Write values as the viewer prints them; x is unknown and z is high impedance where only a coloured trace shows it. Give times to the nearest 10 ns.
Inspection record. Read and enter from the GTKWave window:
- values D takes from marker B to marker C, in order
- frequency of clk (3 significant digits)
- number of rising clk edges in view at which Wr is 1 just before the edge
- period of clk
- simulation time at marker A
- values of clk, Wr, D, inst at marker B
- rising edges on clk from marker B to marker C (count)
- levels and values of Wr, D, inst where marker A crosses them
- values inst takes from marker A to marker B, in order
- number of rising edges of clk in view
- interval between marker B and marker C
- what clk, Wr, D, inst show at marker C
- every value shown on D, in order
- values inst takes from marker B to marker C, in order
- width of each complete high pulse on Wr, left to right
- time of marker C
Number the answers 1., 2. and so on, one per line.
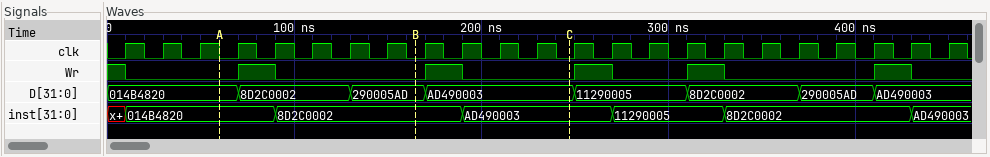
1. 290005AD, AD490003
2. 50.0 MHz
3. 6
4. 20 ns
5. 60 ns
6. clk=0, Wr=0, D=290005AD, inst=8D2C0002
7. 4
8. Wr=0, D=014B4820, inst=014B4820
9. 014B4820, 8D2C0002
10. 23
11. 80 ns
12. clk=0, Wr=0, D=AD490003, inst=AD490003
13. 014B4820, 8D2C0002, 290005AD, AD490003, 11290005, 8D2C0002, 290005AD, AD490003
14. 8D2C0002, AD490003
15. 20 ns, 20 ns, 20 ns, 20 ns, 20 ns
16. 250 ns
